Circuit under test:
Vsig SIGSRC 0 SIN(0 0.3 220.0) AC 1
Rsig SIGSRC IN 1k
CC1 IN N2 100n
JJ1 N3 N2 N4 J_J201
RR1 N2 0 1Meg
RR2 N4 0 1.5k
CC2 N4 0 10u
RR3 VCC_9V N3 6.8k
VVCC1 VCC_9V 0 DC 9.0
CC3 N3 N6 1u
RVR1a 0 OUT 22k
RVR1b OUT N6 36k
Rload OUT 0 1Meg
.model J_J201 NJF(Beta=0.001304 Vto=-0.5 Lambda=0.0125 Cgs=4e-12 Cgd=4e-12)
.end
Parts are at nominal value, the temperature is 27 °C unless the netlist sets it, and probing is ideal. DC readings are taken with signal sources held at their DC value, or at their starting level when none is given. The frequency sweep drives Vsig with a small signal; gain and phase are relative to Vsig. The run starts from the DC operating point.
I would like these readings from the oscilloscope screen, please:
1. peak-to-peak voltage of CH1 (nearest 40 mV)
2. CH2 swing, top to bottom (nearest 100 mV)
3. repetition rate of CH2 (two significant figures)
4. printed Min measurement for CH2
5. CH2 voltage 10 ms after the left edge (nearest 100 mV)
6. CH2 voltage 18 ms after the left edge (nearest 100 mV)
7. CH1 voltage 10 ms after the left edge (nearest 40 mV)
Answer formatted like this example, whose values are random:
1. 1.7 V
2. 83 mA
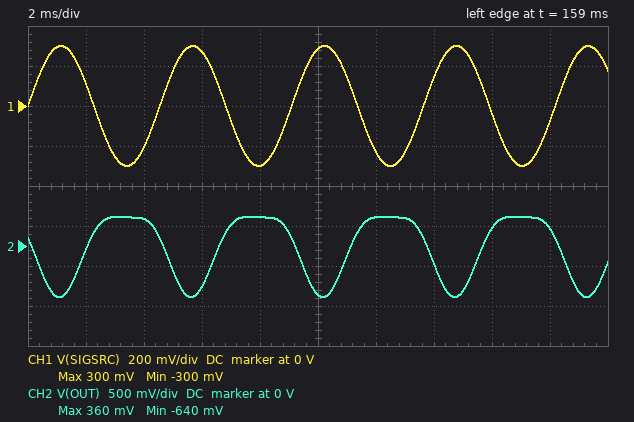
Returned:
1. 600 mV
2. 1.0 V
3. 220 Hz
4. -640 mV
5. -600 mV
6. 200 mV
7. 280 mV
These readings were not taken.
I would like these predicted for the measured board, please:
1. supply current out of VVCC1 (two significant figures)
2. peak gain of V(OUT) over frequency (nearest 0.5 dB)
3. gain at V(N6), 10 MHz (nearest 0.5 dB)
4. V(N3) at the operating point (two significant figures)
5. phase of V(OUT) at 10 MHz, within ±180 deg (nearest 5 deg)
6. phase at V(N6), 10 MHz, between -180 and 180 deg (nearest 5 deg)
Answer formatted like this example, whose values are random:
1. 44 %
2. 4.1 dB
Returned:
1. 130 µA
2. 6.0 dB
3. 10.5 dB
4. 8.1 V
5. 120 deg
6. 120 deg
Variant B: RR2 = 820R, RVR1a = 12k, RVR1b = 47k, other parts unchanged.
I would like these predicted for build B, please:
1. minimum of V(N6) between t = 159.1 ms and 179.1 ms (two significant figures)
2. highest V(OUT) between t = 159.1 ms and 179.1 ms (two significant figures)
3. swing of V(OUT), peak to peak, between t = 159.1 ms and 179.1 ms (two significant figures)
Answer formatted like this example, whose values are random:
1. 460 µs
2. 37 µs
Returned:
1. -2.0 V
2. 260 mV
3. 660 mV
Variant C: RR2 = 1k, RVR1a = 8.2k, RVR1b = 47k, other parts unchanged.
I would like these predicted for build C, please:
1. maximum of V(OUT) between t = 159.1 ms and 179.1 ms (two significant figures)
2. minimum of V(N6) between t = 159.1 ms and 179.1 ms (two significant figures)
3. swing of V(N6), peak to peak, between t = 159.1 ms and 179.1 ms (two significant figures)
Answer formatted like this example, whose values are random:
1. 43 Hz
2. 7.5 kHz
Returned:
1. 170 mV
2. -1.9 V
3. 3.1 V
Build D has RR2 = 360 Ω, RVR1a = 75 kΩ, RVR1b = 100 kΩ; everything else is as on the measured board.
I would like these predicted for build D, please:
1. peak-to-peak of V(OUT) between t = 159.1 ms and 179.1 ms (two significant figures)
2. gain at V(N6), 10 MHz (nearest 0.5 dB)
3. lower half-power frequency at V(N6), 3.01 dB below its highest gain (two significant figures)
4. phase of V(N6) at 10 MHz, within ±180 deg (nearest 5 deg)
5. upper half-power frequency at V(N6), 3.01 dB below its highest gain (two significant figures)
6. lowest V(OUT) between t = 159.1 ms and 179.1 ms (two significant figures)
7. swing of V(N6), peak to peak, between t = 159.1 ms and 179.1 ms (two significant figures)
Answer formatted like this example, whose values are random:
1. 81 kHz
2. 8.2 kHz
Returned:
1. 1.7 V
2. 12.5 dB
3. 11 Hz
4. 115 deg
5. 6.9 MHz
6. -1.1 V
7. 4.2 V
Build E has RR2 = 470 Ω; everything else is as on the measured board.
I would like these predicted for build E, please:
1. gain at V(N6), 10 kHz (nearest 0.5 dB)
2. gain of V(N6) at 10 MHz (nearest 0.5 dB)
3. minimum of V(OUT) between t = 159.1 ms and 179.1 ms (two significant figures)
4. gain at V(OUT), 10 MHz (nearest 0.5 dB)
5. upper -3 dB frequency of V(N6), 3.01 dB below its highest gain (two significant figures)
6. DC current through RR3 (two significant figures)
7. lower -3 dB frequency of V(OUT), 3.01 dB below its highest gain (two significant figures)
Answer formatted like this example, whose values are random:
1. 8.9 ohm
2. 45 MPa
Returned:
1. 16.5 dB
2. 12.0 dB
3. -840 mV
4. 3.5 dB
5. 7.5 MHz
6. 220 µA
7. 21 Hz
